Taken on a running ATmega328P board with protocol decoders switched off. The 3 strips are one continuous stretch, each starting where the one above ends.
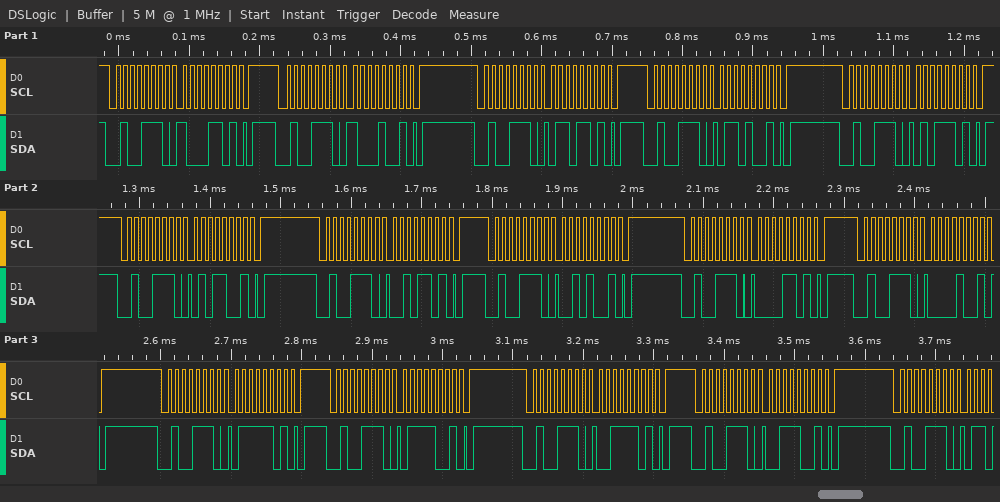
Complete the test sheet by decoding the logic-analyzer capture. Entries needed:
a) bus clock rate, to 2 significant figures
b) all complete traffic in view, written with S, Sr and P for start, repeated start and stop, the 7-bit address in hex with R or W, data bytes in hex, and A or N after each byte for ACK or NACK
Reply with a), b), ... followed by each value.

a) 100 kHz
b) S 27W A 8D A P S 27W A 89 A P S 27W A 6D A P S 27W A 69 A P S 27W A 5D A P S 27W A 59 A P S 27W A 2D A P S 27W A 29 A P S 27W A 0D A P S 27W A 09 A P S 27W A 7D A P S 27W A 79 A P S 27W A 3D A P S 27W A 39 A P S 27W A
